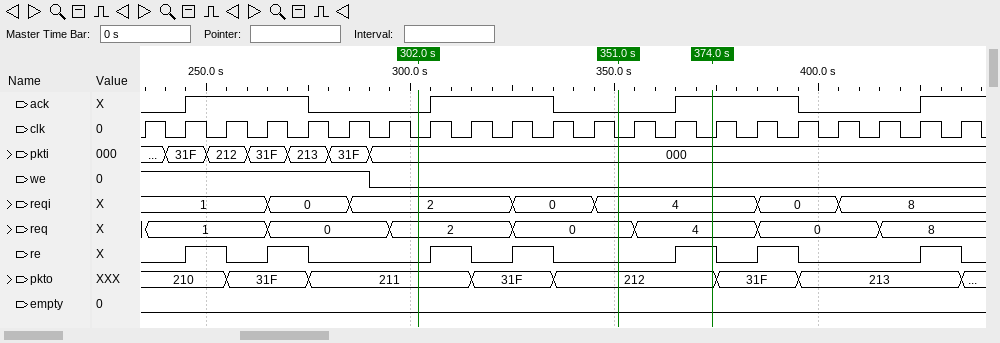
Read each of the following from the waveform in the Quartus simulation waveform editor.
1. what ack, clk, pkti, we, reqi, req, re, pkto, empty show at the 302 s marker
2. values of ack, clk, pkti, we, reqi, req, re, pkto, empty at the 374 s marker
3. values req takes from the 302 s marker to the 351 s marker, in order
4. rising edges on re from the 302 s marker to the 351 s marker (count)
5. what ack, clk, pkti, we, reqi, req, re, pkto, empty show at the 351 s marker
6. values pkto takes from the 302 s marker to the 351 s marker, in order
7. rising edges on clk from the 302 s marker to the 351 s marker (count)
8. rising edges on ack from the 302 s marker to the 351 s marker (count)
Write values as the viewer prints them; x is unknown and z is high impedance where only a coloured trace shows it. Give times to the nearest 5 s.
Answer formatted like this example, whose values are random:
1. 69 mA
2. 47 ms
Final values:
1. ack=0, clk=0, pkti=000, we=0, reqi=2, req=2, re=0, pkto=211, empty=0
2. ack=1, clk=0, pkti=000, we=0, reqi=4, req=4, re=1, pkto=212, empty=0
3. 2, 0
4. 2
5. ack=0, clk=0, pkti=000, we=0, reqi=4, req=0, re=0, pkto=212, empty=0
6. 211, 31F, 212
7. 5
8. 1
